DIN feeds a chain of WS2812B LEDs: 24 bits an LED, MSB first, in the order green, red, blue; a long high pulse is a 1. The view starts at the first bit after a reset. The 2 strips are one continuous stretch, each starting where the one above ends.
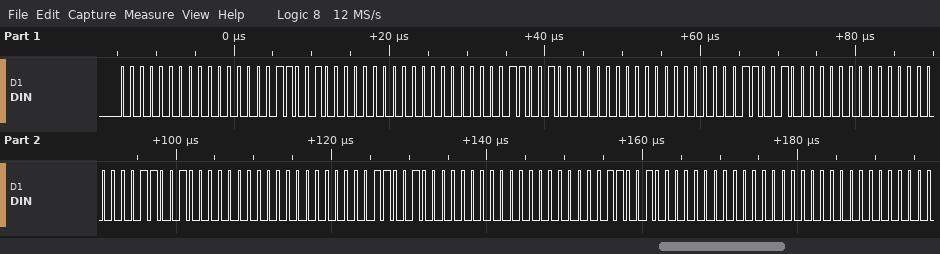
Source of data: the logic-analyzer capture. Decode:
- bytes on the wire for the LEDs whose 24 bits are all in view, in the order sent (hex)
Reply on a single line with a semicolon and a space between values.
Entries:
00 00 C8 00 00 C8 00 00 C8 00 00 C8 00 00 C8 00 00 C8 00 00 00
